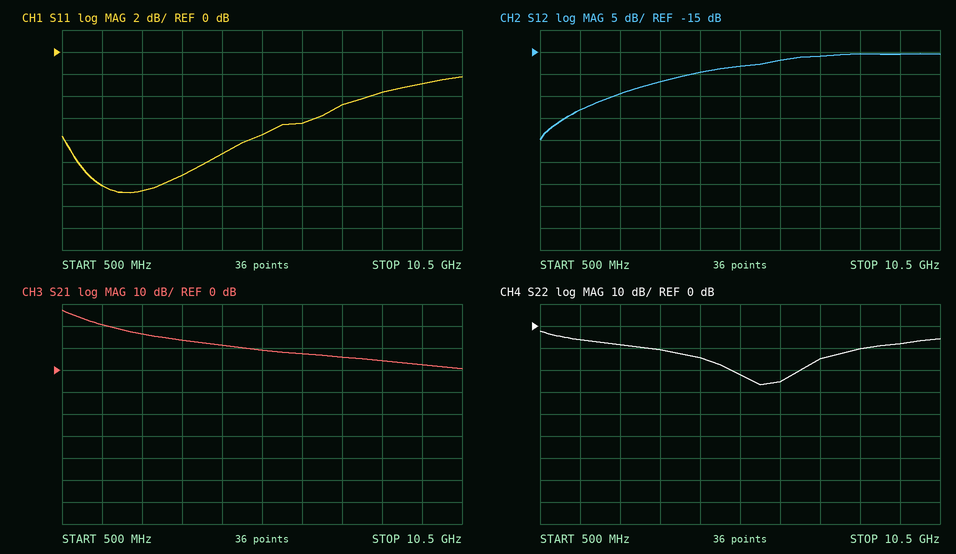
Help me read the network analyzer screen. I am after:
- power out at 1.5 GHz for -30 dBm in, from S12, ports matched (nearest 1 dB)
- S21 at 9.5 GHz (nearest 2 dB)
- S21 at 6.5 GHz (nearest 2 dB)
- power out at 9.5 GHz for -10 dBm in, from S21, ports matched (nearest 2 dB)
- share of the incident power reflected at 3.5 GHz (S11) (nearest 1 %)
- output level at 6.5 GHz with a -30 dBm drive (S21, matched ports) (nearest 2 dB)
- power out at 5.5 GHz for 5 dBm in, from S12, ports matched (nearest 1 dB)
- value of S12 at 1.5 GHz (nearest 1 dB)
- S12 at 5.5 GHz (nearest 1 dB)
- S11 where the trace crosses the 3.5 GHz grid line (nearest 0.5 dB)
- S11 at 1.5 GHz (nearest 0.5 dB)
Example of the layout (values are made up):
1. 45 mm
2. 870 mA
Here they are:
1. -58 dBm
2. 2 dB
3. 8 dB
4. -8 dBm
5. 8 %
6. -22 dBm
7. -13 dBm
8. -28 dB
9. -18 dB
10. -11.0 dB
11. -12.0 dB
